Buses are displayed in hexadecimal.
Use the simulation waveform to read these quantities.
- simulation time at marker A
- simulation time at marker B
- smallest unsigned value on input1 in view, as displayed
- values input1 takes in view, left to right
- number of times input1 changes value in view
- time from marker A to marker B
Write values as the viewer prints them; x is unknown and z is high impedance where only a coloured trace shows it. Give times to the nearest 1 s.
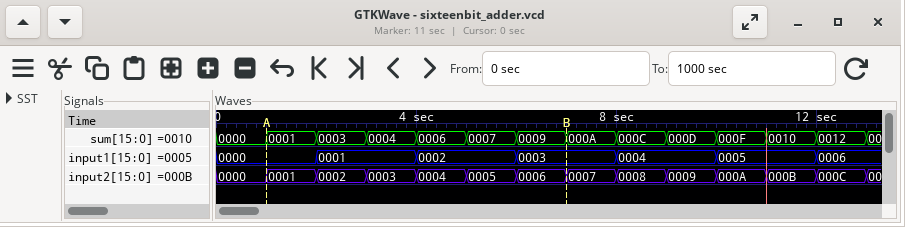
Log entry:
1 s
7 s
0000
0000, 0001, 0002, 0003, 0004, 0005, 0006
6
6 s
